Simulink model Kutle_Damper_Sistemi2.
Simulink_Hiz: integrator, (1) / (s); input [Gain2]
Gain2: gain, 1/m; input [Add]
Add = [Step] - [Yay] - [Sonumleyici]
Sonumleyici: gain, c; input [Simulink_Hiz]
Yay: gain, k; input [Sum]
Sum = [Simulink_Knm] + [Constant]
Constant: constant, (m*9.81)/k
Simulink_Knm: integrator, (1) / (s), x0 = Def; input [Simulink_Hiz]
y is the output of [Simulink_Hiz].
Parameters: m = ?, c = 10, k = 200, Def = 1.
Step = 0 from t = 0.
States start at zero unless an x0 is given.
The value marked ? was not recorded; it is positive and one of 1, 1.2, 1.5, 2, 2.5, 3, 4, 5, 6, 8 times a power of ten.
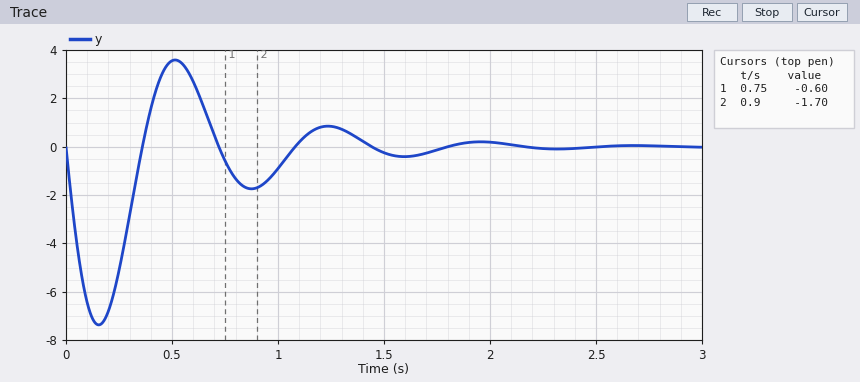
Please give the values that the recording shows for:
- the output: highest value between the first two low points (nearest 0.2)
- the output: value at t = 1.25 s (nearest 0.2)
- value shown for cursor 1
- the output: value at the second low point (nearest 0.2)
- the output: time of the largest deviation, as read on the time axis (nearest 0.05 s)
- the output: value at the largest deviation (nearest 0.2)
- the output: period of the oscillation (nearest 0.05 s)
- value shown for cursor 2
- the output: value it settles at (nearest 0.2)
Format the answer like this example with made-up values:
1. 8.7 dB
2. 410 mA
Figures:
1. 3.6
2. 0.8
3. -0.60
4. -1.8
5. 0.15 s
6. -7.4
7. 0.70 s
8. -1.70
9. 0.0
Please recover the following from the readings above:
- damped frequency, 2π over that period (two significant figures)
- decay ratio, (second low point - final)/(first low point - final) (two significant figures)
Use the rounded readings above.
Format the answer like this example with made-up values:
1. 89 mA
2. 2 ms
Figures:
1. 9.0 rad/s
2. 0.24
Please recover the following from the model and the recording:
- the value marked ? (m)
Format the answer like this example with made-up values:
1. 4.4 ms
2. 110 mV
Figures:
1. 2.5
